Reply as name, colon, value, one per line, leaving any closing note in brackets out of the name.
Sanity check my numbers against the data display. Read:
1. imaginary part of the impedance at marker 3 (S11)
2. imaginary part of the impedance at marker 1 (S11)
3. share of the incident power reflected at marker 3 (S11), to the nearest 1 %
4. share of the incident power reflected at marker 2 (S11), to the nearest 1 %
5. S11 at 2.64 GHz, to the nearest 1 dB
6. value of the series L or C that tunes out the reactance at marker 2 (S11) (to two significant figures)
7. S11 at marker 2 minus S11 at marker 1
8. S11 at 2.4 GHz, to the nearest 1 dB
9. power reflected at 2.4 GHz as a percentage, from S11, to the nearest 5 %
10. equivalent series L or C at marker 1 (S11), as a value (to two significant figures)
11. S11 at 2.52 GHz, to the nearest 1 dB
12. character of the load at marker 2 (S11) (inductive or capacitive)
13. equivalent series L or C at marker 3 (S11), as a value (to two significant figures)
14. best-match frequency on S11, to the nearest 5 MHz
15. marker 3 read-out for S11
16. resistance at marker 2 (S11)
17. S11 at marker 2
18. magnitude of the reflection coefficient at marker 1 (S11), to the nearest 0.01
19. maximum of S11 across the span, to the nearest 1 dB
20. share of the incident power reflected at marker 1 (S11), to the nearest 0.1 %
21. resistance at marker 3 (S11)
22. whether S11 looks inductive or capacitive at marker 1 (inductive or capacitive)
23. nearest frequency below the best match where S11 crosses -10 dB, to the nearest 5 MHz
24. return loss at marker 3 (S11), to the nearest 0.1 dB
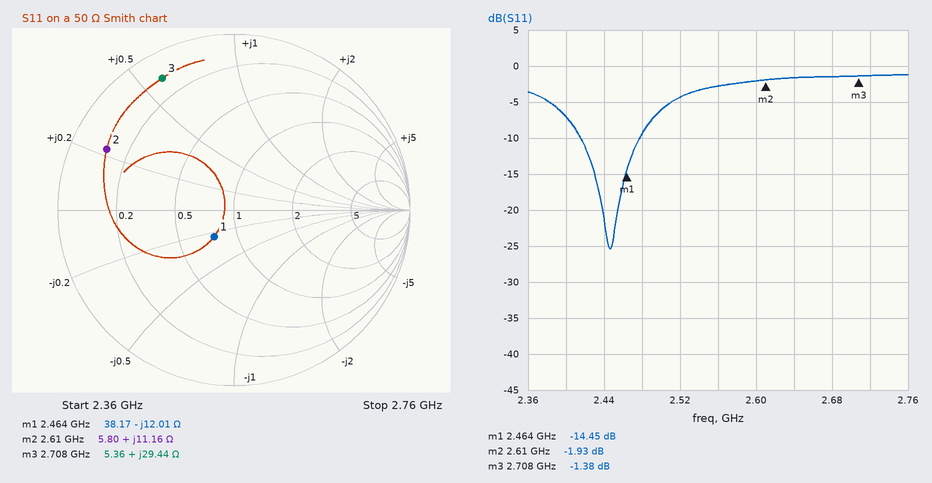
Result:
imaginary part of the impedance at marker 3: +29.44 Ω
imaginary part of the impedance at marker 1: -12.01 Ω
share of the incident power reflected at marker 3 (S11), to the nearest 1 %: 73 %
share of the incident power reflected at marker 2 (S11), to the nearest 1 %: 64 %
S11 at 2.64 GHz, to the nearest 1 dB: -2 dB
value of the series L or C that tunes out the reactance at marker 2 (S11): 5.5 pF
S11 at marker 2 minus S11 at marker 1: 12.52 dB
S11 at 2.4 GHz, to the nearest 1 dB: -7 dB
power reflected at 2.4 GHz as a percentage, from S11, to the nearest 5 %: 20 %
equivalent series L or C at marker 1 (S11), as a value: 5.4 pF
S11 at 2.52 GHz, to the nearest 1 dB: -4 dB
character of the load at marker 2 (S11): inductive
equivalent series L or C at marker 3 (S11), as a value: 1.7 nH
best-match frequency on S11, to the nearest 5 MHz: 2.445 GHz
marker 3 read-out for S11: -1.38 dB
resistance at marker 2: 5.80 Ω
S11 at marker 2: -1.93 dB
magnitude of the reflection coefficient at marker 1 (S11), to the nearest 0.01: 0.19
maximum of S11 across the span, to the nearest 1 dB: -1 dB
share of the incident power reflected at marker 1 (S11), to the nearest 0.1 %: 3.6 %
resistance at marker 3: 5.36 Ω
whether S11 looks inductive or capacitive at marker 1: capacitive
nearest frequency below the best match where S11 crosses -10 dB, to the nearest 5 MHz: 2.415 GHz
return loss at marker 3 (S11), to the nearest 0.1 dB: 1.4 dB
